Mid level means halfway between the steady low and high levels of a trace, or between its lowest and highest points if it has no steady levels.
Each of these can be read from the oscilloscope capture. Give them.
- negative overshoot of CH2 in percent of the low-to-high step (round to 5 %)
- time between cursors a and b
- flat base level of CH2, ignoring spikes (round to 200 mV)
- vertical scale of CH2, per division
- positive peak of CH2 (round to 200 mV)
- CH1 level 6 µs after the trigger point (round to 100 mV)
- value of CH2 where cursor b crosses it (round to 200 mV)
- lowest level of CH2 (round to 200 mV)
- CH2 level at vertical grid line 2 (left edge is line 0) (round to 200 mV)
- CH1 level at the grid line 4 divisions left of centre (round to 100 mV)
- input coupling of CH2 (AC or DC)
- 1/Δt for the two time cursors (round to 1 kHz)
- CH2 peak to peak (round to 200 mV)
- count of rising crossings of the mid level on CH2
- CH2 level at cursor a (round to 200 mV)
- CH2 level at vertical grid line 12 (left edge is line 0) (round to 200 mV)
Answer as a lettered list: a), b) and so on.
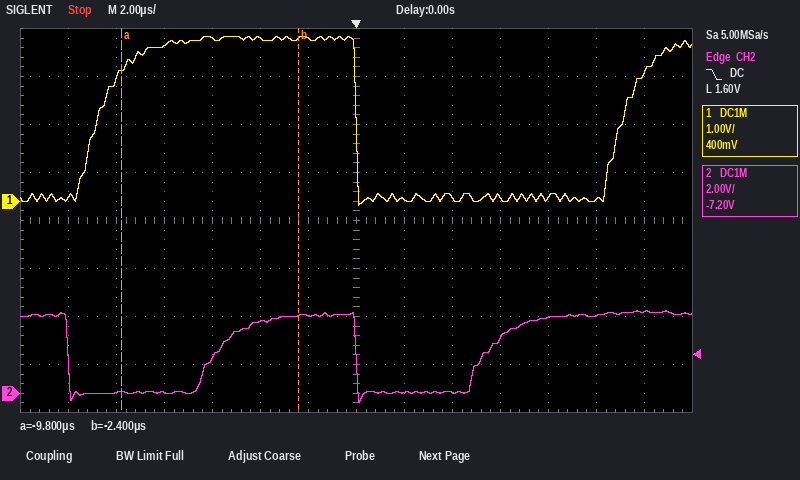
a) 15 %
b) 7.4 µs
c) 0.0 V
d) 2 V
e) 3.4 V
f) 100 mV
g) 3.2 V
h) -400 mV
i) 0.0 V
j) 3.2 V
k) DC
l) 135 kHz
m) 3.8 V
n) 2
o) 0.0 V
p) 3.2 V
